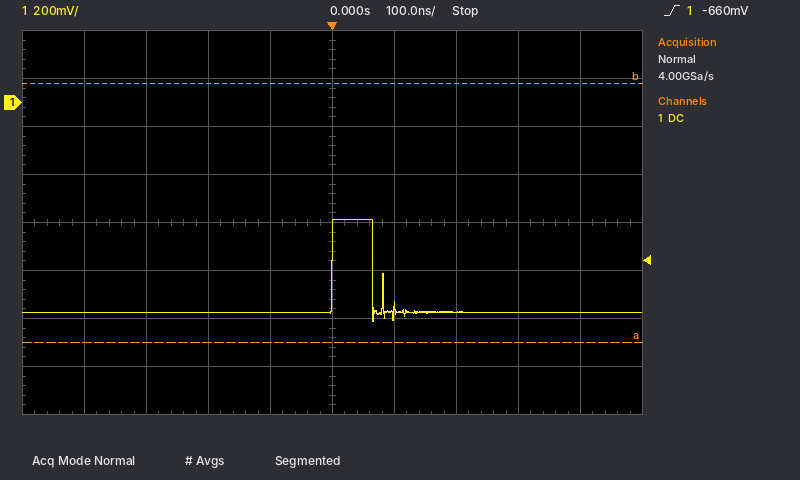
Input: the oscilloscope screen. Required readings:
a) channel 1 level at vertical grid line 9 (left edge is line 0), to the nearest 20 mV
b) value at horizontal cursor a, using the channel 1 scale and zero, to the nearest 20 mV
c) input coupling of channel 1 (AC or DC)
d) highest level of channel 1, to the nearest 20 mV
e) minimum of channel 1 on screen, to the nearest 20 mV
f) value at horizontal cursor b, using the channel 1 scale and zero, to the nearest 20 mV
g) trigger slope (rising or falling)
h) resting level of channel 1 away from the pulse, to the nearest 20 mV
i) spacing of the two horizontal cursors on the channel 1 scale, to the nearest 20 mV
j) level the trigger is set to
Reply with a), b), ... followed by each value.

a) -880 mV
b) -1.00 V
c) DC
d) -480 mV
e) -920 mV
f) 80 mV
g) rising
h) -880 mV
i) 1.08 V
j) -660 mV
